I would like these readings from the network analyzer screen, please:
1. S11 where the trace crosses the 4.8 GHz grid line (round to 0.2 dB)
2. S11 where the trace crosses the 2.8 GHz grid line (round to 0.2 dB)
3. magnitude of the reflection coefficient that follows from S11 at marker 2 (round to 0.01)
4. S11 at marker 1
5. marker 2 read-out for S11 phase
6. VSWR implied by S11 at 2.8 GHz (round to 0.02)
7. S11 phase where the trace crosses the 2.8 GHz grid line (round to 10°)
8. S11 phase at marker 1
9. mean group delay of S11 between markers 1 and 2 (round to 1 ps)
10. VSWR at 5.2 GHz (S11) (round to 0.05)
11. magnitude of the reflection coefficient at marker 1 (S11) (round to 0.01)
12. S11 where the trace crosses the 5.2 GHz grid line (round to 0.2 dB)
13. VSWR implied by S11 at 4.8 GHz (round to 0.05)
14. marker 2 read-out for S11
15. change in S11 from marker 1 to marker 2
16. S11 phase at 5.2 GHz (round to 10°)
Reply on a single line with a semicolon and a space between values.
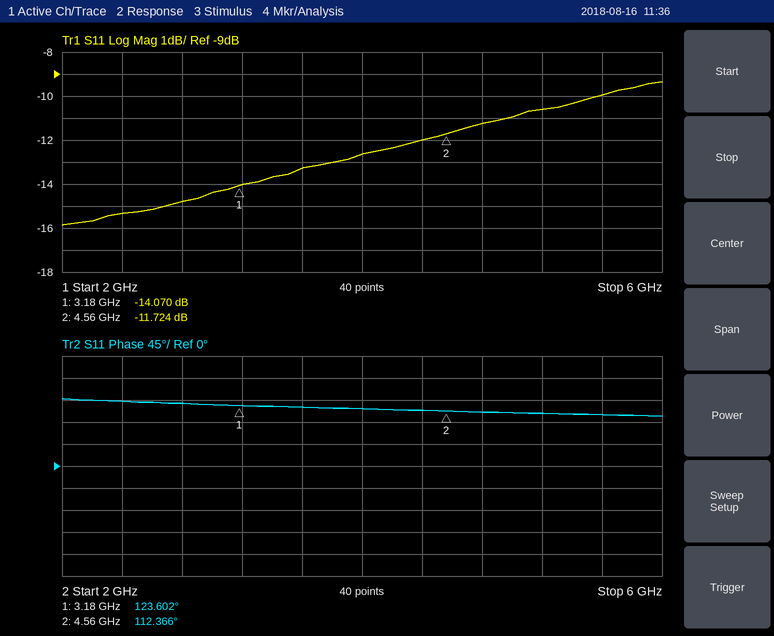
-11.2 dB; -14.8 dB; 0.26; -14.070 dB; 112.366°; 1.44; 130°; 123.602°; 23 ps; 1.85; 0.20; -10.6 dB; 1.75; -11.724 dB; 2.346 dB; 110°
